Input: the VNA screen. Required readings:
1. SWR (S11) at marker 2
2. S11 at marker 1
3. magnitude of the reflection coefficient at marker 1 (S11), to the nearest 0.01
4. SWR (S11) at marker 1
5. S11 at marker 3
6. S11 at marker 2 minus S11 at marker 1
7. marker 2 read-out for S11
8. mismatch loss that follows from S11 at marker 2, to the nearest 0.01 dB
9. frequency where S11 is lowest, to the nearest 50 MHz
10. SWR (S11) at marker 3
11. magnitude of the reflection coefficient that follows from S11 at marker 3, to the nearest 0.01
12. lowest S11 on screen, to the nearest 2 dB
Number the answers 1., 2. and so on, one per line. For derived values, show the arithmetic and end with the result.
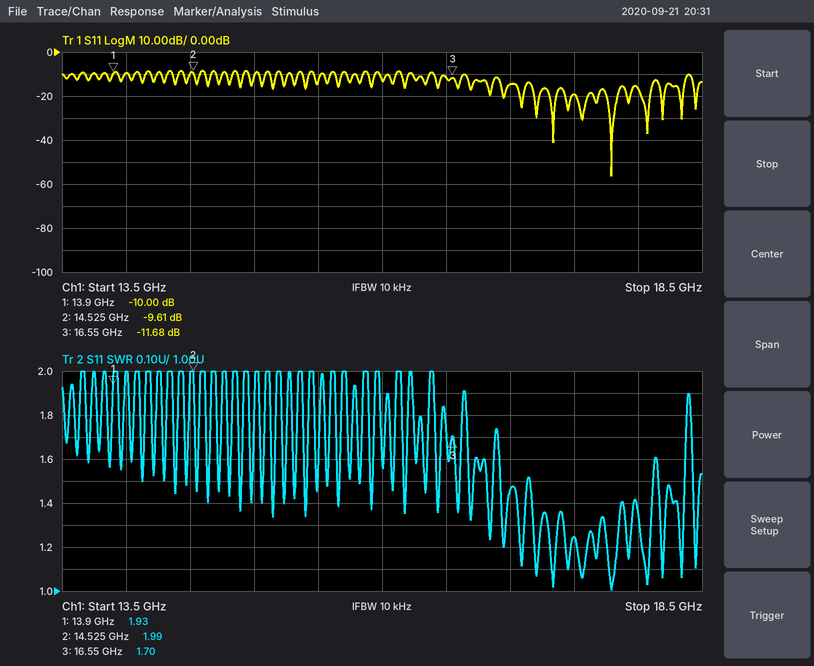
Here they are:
1. 1.99
2. -10.00 dB
3. 10^(-10/20) ≈ 0.32
4. 1.93
5. -11.68 dB
6. -9.61 − (-10) = 0.39 dB
7. -9.61 dB
8. −10 log10(1 − 10^(-9.61/10)) ≈ 0.50 dB
9. 17.80 GHz
10. 1.70
11. 10^(-11.68/20) ≈ 0.26
12. -56 dB
